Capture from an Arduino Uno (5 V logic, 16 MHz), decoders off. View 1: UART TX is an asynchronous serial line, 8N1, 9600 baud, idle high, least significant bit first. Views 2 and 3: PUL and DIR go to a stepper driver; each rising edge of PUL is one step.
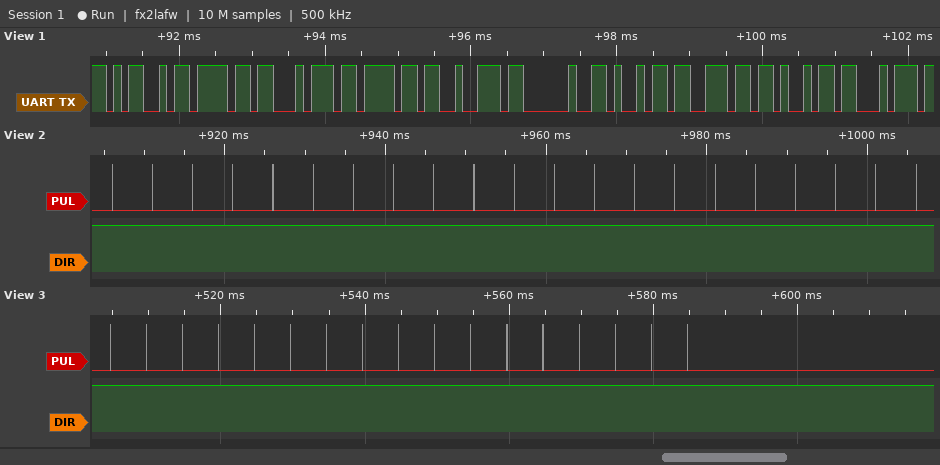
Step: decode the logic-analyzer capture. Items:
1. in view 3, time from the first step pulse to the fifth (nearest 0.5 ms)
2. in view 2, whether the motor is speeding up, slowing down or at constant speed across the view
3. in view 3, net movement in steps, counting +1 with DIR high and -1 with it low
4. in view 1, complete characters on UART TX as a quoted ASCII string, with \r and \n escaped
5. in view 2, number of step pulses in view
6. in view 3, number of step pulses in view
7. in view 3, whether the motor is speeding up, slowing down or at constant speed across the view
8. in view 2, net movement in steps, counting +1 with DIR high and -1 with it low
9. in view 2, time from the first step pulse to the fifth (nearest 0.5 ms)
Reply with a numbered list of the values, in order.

1. 20.0 ms
2. constant speed
3. +17
4. "Motor init"
5. 21
6. 17
7. constant speed
8. +21
9. 20.0 ms
